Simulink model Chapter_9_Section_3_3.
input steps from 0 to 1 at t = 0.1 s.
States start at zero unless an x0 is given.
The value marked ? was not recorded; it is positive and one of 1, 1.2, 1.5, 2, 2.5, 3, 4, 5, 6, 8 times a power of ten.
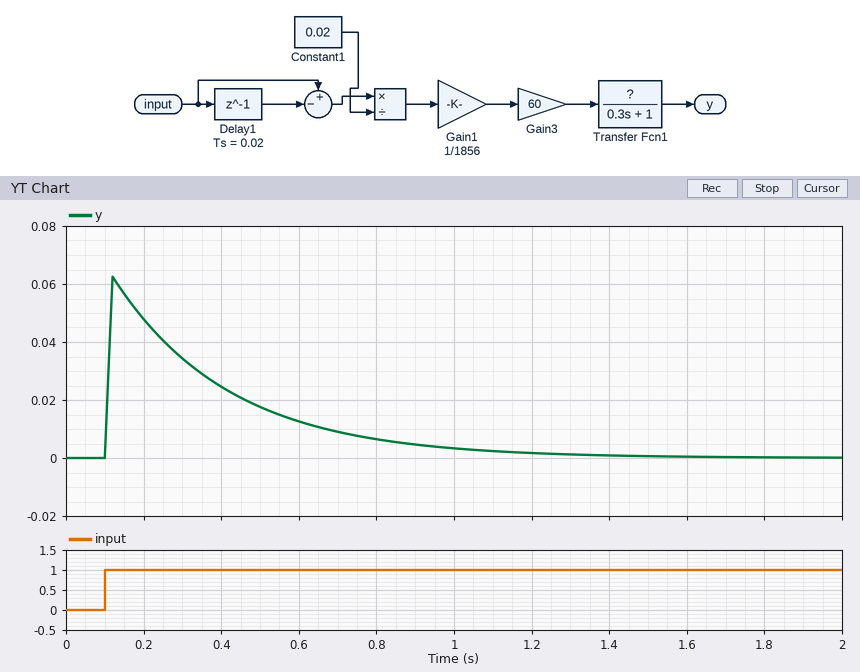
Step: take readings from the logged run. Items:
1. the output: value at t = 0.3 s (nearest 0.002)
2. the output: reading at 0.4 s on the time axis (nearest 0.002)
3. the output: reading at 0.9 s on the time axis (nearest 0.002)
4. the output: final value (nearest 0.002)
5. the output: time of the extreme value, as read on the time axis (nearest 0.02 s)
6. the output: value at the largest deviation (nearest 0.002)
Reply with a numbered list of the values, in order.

1. 0.034
2. 0.024
3. 0.004
4. 0.000
5. 0.12 s
6. 0.062
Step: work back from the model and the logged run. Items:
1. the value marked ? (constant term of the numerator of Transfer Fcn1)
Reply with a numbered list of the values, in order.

1. 0.6
